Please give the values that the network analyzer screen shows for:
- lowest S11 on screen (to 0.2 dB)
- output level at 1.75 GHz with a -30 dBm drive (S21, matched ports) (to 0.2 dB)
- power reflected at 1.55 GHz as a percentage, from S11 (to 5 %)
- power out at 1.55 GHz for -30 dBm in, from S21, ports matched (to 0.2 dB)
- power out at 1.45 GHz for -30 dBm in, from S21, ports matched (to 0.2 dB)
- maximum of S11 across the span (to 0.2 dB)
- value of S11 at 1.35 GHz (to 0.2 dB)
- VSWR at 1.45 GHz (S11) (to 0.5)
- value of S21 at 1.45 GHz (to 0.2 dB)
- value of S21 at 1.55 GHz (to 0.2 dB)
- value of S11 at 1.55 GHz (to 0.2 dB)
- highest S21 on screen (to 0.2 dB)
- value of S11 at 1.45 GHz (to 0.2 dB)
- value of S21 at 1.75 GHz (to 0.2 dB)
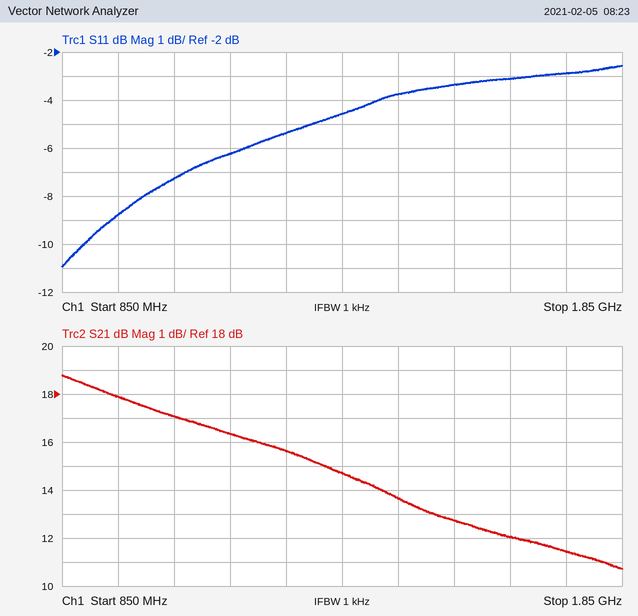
-11.0 dB
-18.6 dBm
45 %
-17.2 dBm
-16.4 dBm
-2.6 dB
-4.6 dB
4.5
13.6 dB
12.8 dB
-3.4 dB
18.8 dB
-3.8 dB
11.4 dB
